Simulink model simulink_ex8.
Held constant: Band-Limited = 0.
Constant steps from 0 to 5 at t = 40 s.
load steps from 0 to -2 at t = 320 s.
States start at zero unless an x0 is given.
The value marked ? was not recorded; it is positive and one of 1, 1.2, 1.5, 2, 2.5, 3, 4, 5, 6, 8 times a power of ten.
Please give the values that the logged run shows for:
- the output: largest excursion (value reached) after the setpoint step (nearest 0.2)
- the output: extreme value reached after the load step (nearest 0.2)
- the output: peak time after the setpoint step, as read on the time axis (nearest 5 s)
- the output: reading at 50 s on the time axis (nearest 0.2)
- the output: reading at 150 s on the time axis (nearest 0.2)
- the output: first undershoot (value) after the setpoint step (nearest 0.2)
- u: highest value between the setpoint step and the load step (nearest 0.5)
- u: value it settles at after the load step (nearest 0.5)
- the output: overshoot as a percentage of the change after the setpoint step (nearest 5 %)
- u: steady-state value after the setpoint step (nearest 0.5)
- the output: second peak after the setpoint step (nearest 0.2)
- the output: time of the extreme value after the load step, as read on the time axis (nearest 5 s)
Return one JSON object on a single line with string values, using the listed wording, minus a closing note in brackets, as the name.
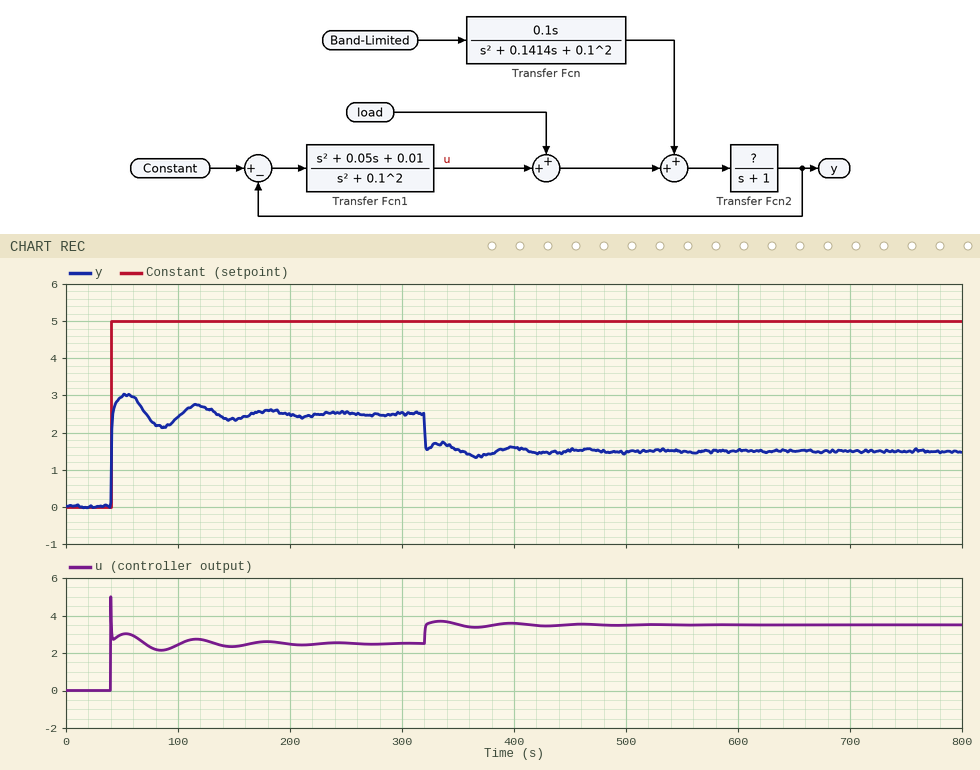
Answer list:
{"the output: largest excursion (value reached) after the setpoint step": "3.0", "the output: extreme value reached after the load step": "1.4", "the output: peak time after the setpoint step, as read on the time axis": "55 s", "the output: reading at 50 s on the time axis": "3.0", "the output: reading at 150 s on the time axis": "2.4", "the output: first undershoot (value) after the setpoint step": "2.2", "u: highest value between the setpoint step and the load step": "5.0", "u: value it settles at after the load step": "3.5", "the output: overshoot as a percentage of the change after the setpoint step": "20 %", "u: steady-state value after the setpoint step": "2.5", "the output: second peak after the setpoint step": "2.8", "the output: time of the extreme value after the load step, as read on the time axis": "365 s"}
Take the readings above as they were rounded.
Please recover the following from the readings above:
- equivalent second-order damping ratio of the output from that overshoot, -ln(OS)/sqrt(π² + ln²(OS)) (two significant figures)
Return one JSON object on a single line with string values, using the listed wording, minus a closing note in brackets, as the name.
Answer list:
{"equivalent second-order damping ratio of the output from that overshoot, -ln(OS)/sqrt(π² + ln²(OS))": "0.46"}
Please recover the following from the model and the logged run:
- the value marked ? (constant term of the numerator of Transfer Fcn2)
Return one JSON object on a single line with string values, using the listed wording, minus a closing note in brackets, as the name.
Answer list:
{"the value marked ?": "1"}
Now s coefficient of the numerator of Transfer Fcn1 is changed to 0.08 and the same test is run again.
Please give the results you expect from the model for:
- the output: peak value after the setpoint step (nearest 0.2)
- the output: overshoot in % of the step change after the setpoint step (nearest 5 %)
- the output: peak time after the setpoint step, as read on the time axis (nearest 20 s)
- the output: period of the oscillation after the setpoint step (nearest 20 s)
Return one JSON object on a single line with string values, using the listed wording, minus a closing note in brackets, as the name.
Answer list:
{"the output: peak value after the setpoint step": "3.2", "the output: overshoot in % of the step change after the setpoint step": "30 %", "the output: peak time after the setpoint step, as read on the time axis": "60 s", "the output: period of the oscillation after the setpoint step": "60 s"}
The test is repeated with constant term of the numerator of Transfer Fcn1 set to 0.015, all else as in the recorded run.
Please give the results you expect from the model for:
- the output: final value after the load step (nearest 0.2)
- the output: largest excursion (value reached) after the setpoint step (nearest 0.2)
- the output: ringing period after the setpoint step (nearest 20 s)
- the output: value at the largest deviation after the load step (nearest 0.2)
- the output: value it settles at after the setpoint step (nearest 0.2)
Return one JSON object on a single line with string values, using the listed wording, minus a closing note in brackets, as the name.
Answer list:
{"the output: final value after the load step": "2.2", "the output: largest excursion (value reached) after the setpoint step": "3.6", "the output: ringing period after the setpoint step": "60 s", "the output: value at the largest deviation after the load step": "2.0", "the output: value it settles at after the setpoint step": "3.0"}
